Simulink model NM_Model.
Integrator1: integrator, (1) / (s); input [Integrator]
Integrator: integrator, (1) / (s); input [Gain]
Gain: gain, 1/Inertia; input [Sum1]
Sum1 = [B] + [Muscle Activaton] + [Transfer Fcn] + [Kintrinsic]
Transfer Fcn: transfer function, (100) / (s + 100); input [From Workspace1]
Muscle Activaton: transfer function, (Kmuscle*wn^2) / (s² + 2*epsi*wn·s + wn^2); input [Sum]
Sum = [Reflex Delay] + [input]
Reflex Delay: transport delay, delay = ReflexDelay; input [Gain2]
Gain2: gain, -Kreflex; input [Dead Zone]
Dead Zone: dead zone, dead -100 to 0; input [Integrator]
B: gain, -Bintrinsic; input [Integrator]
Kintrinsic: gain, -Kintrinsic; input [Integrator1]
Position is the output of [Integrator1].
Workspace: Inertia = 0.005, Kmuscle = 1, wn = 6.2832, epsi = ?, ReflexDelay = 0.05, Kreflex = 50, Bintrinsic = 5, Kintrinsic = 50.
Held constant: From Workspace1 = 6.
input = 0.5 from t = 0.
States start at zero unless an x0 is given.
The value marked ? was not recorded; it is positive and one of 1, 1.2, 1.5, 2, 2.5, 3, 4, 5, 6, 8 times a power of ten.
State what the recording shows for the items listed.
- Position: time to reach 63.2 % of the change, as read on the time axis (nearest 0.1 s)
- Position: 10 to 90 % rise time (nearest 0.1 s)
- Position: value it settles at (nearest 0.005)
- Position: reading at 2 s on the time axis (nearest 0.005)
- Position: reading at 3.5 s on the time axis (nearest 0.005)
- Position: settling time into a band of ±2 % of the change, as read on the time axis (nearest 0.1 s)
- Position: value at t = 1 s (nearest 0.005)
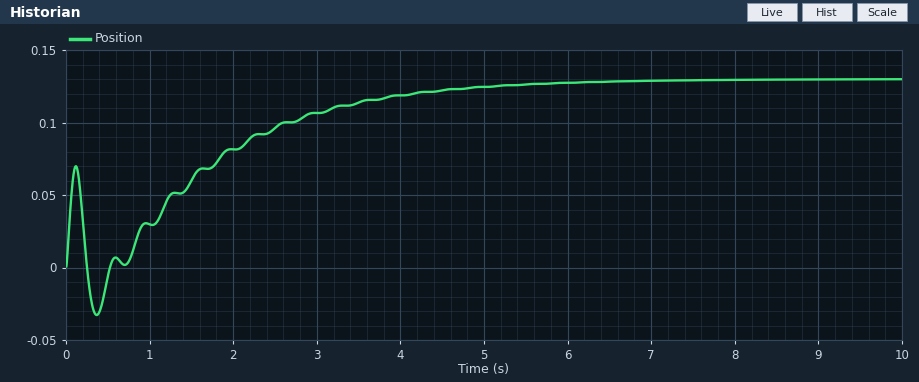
2.1 s
3.8 s
0.130
0.080
0.115
6.1 s
0.030
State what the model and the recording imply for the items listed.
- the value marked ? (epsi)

0.8
